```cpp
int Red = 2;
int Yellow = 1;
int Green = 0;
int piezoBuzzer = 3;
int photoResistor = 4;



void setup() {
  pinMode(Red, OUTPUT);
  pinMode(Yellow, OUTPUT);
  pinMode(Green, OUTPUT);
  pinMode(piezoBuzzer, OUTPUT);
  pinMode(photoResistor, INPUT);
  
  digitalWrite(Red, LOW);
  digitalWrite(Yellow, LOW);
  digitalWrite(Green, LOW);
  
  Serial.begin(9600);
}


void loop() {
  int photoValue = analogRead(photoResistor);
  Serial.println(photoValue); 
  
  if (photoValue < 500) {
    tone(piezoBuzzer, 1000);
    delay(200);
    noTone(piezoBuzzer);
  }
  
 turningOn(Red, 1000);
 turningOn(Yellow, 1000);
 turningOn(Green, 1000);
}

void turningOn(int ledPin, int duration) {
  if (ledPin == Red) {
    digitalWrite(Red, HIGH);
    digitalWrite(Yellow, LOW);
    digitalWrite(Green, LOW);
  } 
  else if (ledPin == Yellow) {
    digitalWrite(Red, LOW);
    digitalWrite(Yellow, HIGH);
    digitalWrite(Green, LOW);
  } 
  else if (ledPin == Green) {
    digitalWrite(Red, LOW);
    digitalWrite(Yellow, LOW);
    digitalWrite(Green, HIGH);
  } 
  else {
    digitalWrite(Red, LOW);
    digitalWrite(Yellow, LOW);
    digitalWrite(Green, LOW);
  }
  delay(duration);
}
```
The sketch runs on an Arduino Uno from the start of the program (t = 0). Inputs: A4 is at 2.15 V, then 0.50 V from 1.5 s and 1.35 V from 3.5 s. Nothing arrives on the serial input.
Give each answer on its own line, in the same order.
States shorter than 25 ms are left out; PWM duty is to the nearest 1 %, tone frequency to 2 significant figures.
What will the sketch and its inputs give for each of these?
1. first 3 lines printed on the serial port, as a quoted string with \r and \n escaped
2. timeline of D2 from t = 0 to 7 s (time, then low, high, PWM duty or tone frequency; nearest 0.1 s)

"440\r\n102\r\n276\r\n"
0 s low; 0.2 s high; 1.2 s low; 3.4 s high; 4.4 s low; 6.6 s high
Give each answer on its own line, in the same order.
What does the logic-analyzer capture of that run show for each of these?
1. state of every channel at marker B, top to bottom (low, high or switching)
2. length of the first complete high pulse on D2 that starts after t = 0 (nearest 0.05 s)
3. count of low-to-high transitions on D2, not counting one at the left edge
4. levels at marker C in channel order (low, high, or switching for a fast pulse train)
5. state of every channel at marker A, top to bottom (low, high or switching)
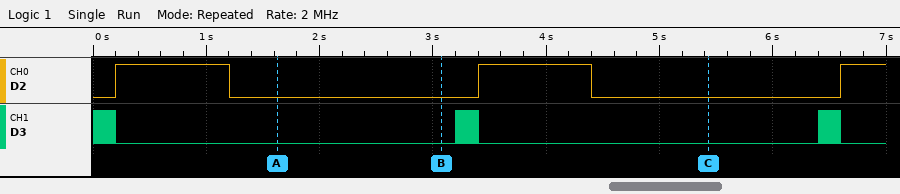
D2 low, D3 low
1.00 s
3
D2 low, D3 low
D2 low, D3 low
